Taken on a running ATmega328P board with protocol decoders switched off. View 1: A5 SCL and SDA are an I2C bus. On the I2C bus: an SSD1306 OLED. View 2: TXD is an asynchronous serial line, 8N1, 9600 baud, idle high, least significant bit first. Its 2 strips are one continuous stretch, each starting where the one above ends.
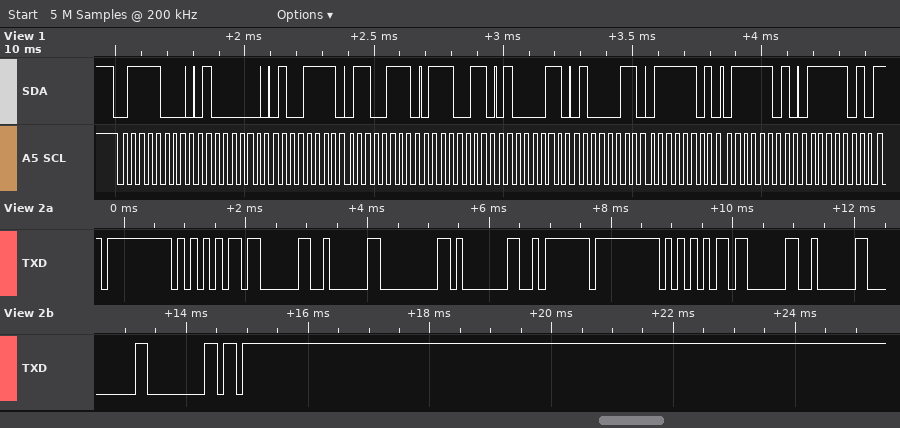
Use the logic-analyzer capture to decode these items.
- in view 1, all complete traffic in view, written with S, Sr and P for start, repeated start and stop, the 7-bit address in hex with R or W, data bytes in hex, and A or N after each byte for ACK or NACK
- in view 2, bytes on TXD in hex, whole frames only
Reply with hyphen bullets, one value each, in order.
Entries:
- S 3CW A 40 A 4F A 67 A 73 A 43 A 43 A 7D A 7D A 7D A
- FF 55 03 02 00 01 FA FF 55 03 02 00 00 FB
